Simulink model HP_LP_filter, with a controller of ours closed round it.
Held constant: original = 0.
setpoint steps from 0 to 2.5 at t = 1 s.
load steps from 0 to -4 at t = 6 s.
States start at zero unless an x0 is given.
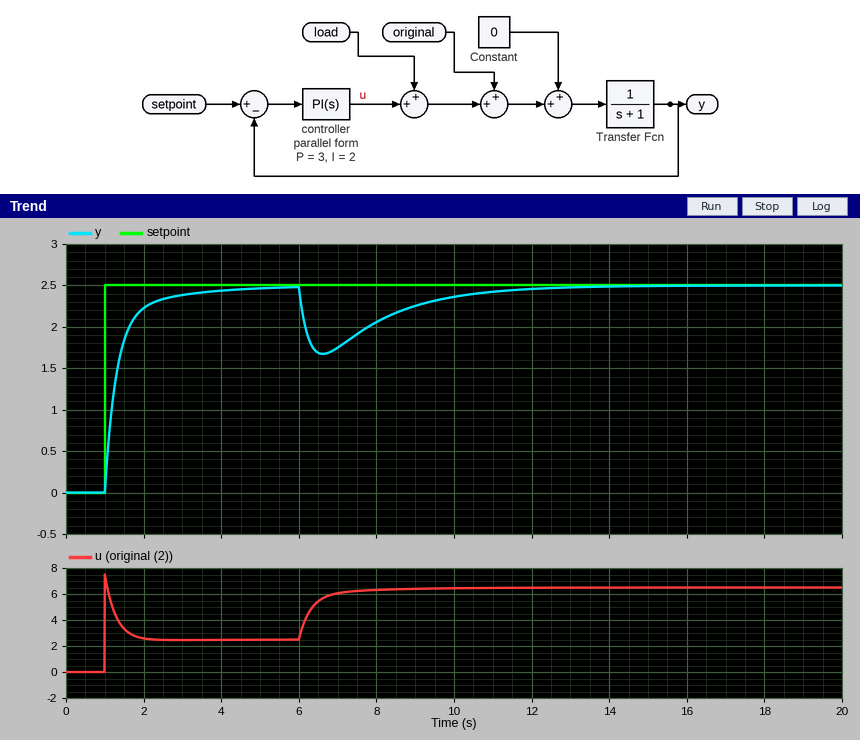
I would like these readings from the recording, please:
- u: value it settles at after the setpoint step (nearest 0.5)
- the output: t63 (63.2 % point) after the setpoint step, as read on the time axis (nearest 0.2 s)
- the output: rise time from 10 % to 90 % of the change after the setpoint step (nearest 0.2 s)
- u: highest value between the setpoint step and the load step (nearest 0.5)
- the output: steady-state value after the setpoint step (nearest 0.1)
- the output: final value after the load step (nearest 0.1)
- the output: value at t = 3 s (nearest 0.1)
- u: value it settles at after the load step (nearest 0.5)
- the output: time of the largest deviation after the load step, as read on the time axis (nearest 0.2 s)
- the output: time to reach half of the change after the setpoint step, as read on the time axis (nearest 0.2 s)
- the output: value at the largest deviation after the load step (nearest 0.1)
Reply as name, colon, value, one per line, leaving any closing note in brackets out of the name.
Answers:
u: value it settles at after the setpoint step: 2.5
the output: t63 (63.2 % point) after the setpoint step, as read on the time axis: 1.4 s
the output: rise time from 10 % to 90 % of the change after the setpoint step: 1.0 s
u: highest value between the setpoint step and the load step: 7.5
the output: steady-state value after the setpoint step: 2.5
the output: final value after the load step: 2.5
the output: value at t = 3 s: 2.4
u: value it settles at after the load step: 6.5
the output: time of the largest deviation after the load step, as read on the time axis: 6.6 s
the output: time to reach half of the change after the setpoint step, as read on the time axis: 1.2 s
the output: value at the largest deviation after the load step: 1.7
